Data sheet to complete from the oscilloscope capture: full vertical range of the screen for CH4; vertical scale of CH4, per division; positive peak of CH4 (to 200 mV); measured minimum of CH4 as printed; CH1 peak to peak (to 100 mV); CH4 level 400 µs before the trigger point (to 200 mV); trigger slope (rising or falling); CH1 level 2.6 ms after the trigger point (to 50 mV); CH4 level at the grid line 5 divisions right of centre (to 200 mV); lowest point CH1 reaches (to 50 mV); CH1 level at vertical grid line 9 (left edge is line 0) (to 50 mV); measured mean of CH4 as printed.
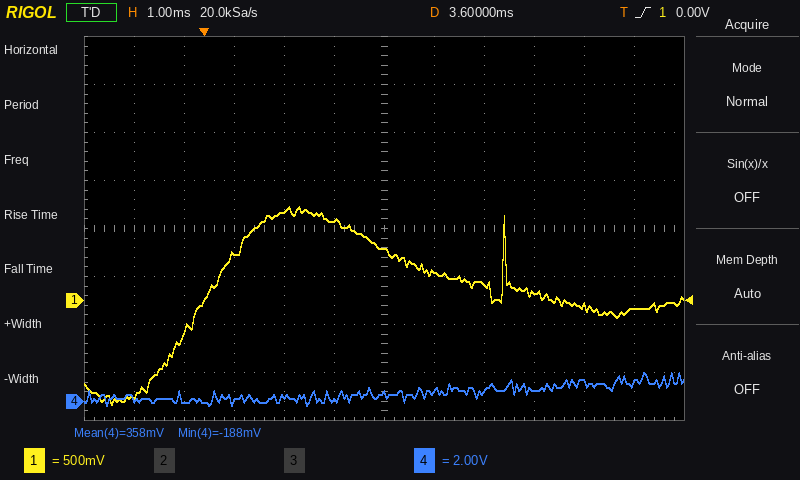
16 V
2 V
1.2 V
-188 mV
2.10 V
0.0 V
rising
850 mV
800 mV
-1.10 V
100 mV
358 mV
